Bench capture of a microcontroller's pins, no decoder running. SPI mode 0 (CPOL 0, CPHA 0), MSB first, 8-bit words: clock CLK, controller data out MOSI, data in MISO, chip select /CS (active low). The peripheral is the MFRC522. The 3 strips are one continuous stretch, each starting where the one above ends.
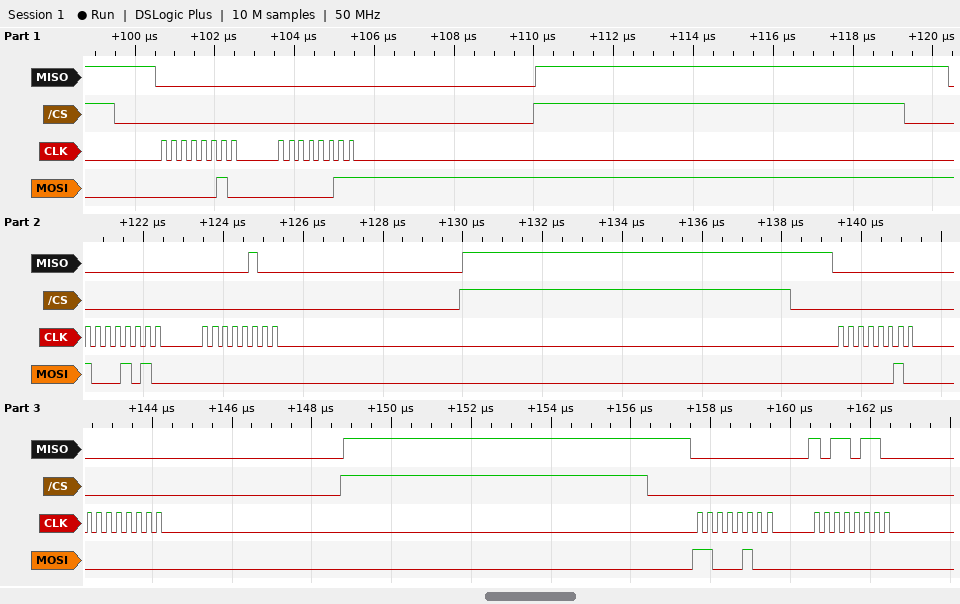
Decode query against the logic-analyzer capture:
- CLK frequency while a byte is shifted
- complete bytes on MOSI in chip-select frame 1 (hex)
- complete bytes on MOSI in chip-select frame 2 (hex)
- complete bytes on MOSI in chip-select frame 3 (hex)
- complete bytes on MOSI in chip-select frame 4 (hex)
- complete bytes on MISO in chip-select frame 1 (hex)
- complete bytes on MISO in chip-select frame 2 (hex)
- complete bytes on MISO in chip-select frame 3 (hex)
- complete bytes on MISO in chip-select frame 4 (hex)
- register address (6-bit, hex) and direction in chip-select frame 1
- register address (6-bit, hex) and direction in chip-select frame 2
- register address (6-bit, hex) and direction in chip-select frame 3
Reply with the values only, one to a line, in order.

4 MHz
02 03
8A 00
02 00
C4 00
00 00
00 04
00 00
00 B6
0x01 write
0x05 read
0x01 write
